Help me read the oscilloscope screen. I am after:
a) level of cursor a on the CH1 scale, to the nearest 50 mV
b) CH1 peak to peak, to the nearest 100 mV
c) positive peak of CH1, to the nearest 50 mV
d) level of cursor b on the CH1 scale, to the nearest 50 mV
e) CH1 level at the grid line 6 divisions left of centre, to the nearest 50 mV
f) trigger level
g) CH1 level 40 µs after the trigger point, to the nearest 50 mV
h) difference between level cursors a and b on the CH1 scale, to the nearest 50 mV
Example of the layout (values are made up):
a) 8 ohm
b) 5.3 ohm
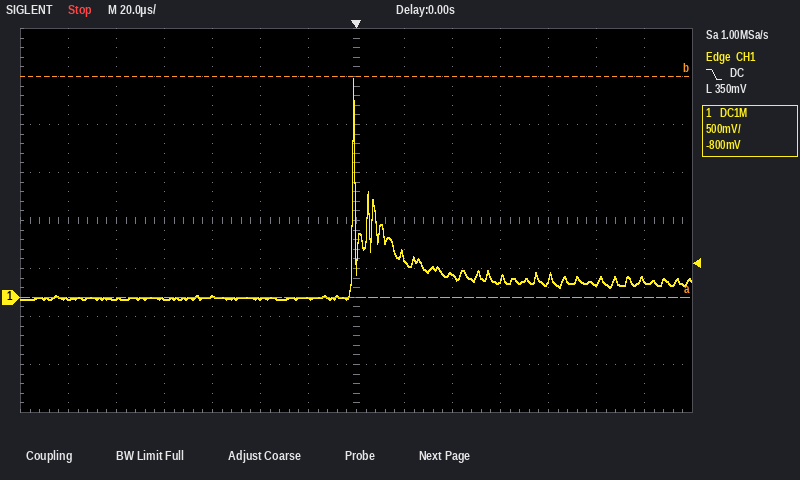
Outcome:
a) 0 mV
b) 2.30 V
c) 2.30 V
d) 2.30 V
e) 0 mV
f) 350 mV
g) 250 mV
h) 2.30 V
